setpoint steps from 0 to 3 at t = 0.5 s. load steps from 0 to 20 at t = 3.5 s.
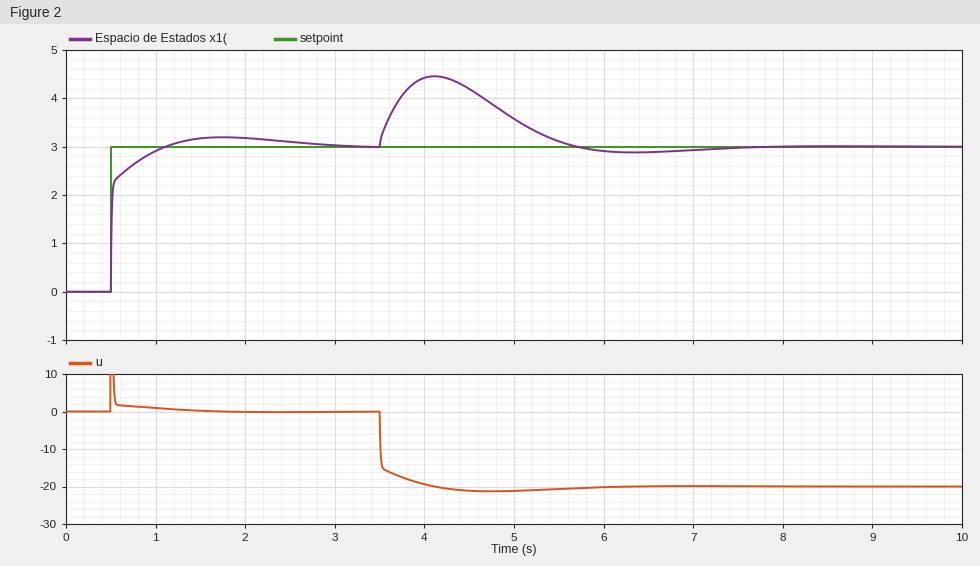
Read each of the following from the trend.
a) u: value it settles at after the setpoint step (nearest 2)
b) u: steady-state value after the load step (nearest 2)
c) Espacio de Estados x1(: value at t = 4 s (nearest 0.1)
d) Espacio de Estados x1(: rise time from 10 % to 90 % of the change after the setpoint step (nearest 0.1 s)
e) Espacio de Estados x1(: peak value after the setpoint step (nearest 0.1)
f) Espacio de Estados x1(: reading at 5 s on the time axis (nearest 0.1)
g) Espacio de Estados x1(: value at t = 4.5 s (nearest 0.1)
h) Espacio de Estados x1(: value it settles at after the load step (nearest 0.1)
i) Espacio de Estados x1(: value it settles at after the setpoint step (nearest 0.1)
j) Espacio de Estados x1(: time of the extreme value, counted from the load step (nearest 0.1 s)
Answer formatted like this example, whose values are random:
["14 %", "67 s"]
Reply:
["0", "-20", "4.4", "0.3 s", "3.2", "3.6", "4.2", "3.0", "3.0", "0.6 s"]
